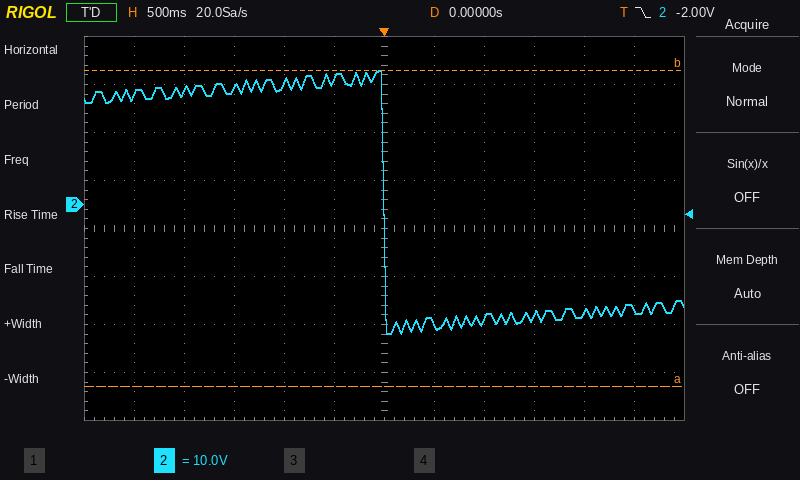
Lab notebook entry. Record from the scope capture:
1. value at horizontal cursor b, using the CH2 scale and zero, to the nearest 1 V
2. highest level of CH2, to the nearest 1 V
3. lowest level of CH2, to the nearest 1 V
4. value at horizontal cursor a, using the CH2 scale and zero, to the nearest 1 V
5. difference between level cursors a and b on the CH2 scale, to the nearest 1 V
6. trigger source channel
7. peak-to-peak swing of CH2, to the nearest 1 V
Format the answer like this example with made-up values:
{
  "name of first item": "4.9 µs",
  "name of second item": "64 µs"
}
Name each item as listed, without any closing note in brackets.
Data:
{
  "value at horizontal cursor b, using the CH2 scale and zero, to the nearest 1 V": "28 V",
  "highest level of CH2, to the nearest 1 V": "28 V",
  "lowest level of CH2, to the nearest 1 V": "-27 V",
  "value at horizontal cursor a, using the CH2 scale and zero, to the nearest 1 V": "-38 V",
  "difference between level cursors a and b on the CH2 scale, to the nearest 1 V": "66 V",
  "trigger source channel": "CH2",
  "peak-to-peak swing of CH2, to the nearest 1 V": "55 V"
}
